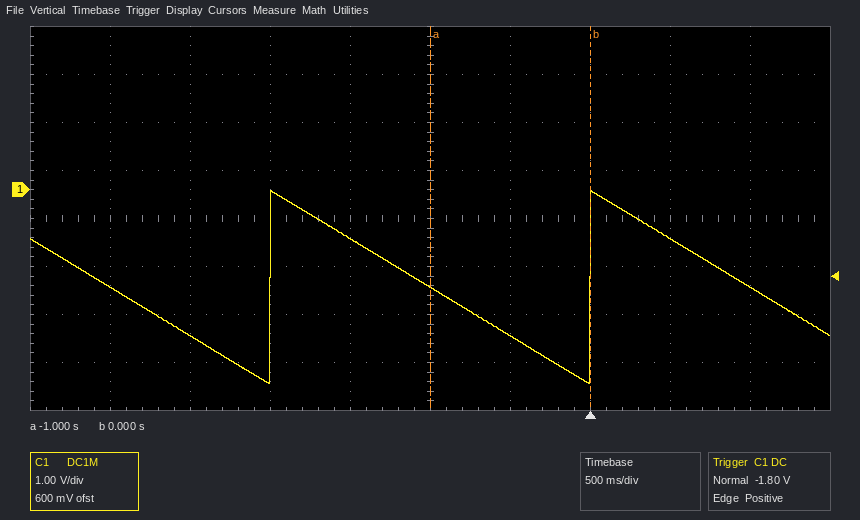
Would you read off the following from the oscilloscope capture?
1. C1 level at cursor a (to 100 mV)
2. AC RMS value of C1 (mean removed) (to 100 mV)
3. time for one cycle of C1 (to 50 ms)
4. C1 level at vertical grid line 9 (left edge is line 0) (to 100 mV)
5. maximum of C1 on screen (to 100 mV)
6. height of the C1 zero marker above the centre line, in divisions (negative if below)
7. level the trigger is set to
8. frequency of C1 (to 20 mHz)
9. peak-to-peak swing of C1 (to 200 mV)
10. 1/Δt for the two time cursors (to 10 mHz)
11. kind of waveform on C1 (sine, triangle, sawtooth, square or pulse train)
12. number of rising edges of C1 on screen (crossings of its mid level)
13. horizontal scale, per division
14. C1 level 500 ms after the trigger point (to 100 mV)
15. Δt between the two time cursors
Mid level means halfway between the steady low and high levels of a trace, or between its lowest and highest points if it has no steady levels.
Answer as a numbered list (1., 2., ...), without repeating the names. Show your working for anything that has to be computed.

1. -2.0 V
2. 4.0 V / (2√3) ≈ 1.2 V
3. 2.00 s
4. -2.0 V
5. 0.0 V
6. +0.6 div
7. -1.80 V
8. 1 / 2.00 s ≈ 500 mHz
9. 4.0 V
10. 1 / 1.00 s ≈ 1.00 Hz
11. sawtooth
12. 2
13. 500 ms
14. -1.0 V
15. 0 s − (-1 s) = 1.00 s
